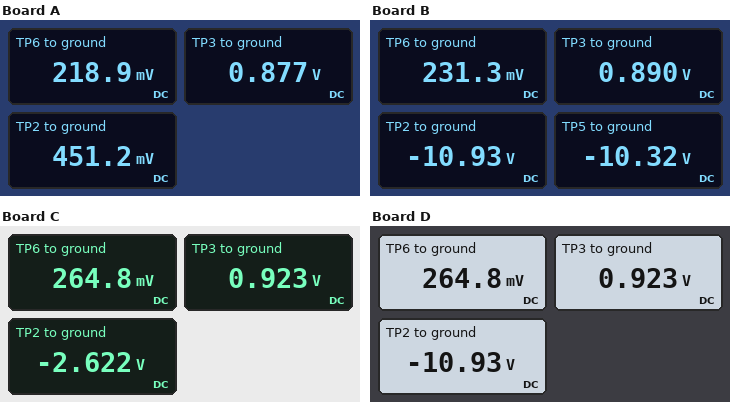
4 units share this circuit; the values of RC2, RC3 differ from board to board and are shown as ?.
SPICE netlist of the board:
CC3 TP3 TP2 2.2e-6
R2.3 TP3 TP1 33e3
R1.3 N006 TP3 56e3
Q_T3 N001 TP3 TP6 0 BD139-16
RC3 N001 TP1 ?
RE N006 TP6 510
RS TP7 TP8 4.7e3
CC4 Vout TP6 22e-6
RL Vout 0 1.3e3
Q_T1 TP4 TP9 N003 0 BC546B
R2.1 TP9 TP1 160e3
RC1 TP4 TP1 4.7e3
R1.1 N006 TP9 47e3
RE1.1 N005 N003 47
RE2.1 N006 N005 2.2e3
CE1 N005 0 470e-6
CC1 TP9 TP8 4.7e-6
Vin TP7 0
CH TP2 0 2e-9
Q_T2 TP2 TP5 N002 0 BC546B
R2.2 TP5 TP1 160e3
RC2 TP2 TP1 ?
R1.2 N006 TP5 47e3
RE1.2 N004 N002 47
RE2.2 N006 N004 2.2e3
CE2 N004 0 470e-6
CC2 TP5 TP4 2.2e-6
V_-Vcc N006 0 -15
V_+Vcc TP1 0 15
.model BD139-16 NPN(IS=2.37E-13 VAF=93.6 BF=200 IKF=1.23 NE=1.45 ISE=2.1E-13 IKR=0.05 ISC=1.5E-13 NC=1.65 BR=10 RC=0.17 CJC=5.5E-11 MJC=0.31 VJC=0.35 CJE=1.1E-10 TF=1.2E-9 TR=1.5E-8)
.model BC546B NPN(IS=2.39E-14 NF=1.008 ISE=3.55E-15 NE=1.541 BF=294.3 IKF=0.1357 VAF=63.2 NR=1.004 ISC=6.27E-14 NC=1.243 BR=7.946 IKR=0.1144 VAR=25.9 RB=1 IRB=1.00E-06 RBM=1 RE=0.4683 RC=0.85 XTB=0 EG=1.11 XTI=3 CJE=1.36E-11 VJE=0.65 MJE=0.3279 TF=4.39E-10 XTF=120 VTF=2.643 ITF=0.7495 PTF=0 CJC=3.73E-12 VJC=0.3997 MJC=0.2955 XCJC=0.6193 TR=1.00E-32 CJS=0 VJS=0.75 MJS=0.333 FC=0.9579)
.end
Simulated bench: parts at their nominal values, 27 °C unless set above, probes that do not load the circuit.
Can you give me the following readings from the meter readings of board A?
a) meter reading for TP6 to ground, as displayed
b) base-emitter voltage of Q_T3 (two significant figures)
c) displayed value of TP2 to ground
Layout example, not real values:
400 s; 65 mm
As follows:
218.9 mV; 660 mV; 451.2 mV
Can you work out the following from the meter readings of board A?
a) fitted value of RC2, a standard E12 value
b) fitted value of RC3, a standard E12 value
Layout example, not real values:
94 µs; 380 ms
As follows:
5.6 kΩ; 100 Ω
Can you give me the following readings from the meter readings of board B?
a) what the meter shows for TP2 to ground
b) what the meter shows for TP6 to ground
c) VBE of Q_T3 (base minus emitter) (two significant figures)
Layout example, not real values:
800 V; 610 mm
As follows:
-10.93 V; 231.3 mV; 660 mV
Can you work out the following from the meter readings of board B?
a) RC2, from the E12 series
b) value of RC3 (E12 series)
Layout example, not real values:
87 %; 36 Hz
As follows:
15 kΩ; 82 Ω
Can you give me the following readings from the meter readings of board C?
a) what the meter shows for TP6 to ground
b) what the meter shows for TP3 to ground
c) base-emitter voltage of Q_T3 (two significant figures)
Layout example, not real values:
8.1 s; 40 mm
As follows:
264.8 mV; 0.923 V; 660 mV
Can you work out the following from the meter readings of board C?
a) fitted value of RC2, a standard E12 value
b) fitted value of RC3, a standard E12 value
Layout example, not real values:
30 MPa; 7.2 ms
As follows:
6.8 kΩ; 33 Ω
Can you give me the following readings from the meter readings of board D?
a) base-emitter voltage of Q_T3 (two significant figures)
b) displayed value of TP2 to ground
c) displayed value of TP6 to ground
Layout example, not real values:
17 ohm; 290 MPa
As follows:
660 mV; -10.93 V; 264.8 mV
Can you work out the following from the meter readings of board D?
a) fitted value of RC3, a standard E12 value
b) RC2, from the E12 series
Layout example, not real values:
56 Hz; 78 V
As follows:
33 Ω; 15 kΩ
